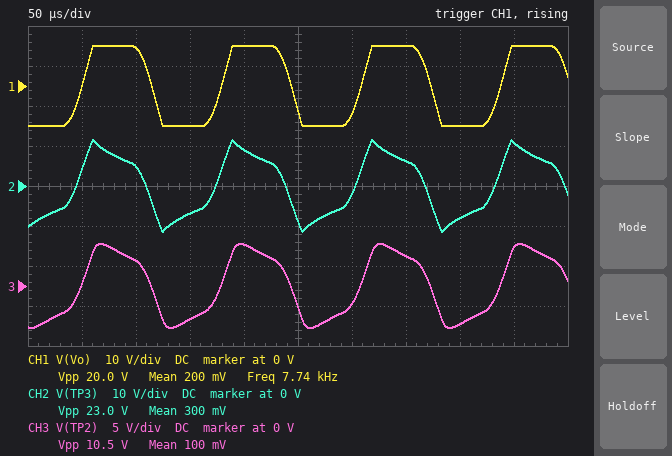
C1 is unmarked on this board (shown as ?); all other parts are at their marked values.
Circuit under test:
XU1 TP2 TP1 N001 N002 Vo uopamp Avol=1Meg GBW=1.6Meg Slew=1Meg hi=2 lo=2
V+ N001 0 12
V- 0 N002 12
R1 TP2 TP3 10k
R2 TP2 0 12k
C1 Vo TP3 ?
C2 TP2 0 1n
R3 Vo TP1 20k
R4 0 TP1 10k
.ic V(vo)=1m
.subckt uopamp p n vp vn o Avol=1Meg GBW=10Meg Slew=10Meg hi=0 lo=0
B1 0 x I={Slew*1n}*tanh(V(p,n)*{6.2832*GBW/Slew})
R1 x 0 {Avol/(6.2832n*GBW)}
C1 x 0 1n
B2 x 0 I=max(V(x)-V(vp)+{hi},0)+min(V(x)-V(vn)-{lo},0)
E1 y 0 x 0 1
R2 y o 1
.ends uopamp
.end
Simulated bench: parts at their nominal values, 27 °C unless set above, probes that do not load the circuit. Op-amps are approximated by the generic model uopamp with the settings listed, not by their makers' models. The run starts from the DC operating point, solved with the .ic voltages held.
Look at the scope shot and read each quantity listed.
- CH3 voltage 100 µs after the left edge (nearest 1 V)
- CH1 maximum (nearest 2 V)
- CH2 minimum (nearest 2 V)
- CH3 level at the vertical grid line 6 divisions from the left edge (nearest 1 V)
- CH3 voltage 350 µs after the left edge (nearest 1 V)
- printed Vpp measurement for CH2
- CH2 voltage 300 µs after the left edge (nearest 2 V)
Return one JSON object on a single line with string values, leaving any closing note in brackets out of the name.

{"CH3 voltage 100 µs after the left edge": "3 V", "CH1 maximum": "10 V", "CH2 minimum": "-12 V", "CH3 level at the vertical grid line 6 divisions from the left edge": "-2 V", "CH3 voltage 350 µs after the left edge": "4 V", "printed Vpp measurement for CH2": "23.0 V", "CH2 voltage 300 µs after the left edge": "-2 V"}
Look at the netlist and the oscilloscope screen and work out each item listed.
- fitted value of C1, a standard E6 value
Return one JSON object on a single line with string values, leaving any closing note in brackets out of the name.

{"fitted value of C1, a standard E6 value": "2.2 nF"}
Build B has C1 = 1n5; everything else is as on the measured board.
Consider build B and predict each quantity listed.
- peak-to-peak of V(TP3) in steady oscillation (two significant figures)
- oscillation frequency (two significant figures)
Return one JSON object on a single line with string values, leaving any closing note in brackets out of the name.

{"peak-to-peak of V(TP3) in steady oscillation": "21 V", "oscillation frequency": "10 kHz"}
